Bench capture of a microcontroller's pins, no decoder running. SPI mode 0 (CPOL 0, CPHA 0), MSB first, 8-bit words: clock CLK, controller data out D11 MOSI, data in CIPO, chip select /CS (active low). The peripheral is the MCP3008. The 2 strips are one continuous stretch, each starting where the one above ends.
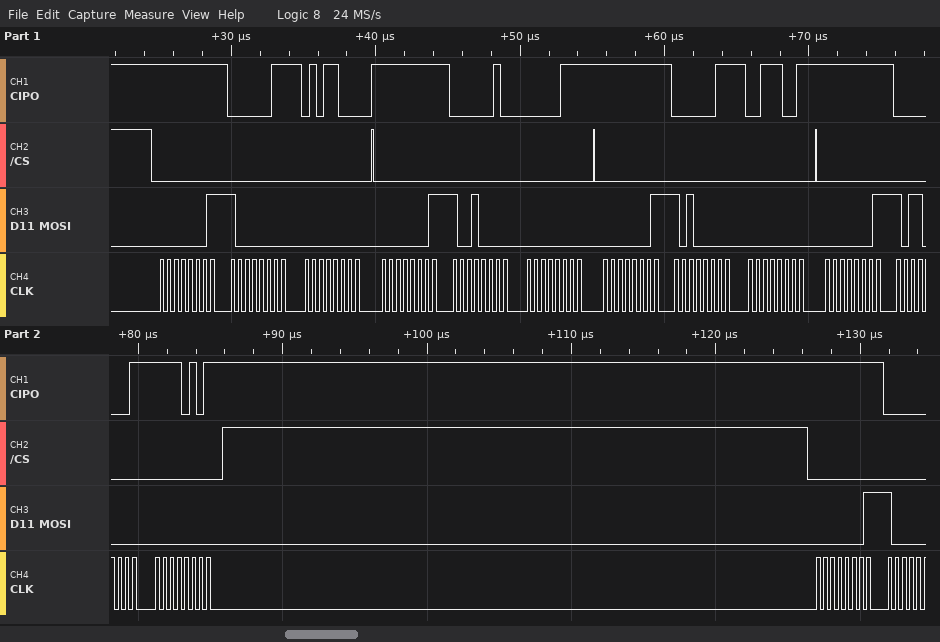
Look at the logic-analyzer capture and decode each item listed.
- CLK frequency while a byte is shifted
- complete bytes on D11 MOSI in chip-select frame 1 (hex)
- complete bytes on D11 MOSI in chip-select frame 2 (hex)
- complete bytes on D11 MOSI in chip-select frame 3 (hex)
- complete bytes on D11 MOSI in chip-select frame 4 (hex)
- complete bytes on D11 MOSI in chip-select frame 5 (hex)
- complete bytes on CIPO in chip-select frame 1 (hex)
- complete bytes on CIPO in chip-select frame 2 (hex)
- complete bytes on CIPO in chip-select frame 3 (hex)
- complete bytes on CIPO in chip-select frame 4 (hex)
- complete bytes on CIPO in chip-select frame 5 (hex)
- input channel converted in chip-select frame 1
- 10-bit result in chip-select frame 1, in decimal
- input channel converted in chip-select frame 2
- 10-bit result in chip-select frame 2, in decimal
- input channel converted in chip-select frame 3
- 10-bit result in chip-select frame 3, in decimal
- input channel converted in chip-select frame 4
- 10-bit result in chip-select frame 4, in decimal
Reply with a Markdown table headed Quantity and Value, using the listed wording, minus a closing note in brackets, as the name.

| Quantity | Value |
|---|---|
| CLK frequency while a byte is shifted | 2 MHz |
| complete bytes on D11 MOSI in chip-select frame 1 | 01 80 00 |
| complete bytes on D11 MOSI in chip-select frame 2 | 01 90 00 |
| complete bytes on D11 MOSI in chip-select frame 3 | 01 A0 00 |
| complete bytes on D11 MOSI in chip-select frame 4 | 01 B0 00 |
| complete bytes on D11 MOSI in chip-select frame 5 | 01 |
| complete bytes on CIPO in chip-select frame 1 | FF 03 58 |
| complete bytes on CIPO in chip-select frame 2 | FF 02 07 |
| complete bytes on CIPO in chip-select frame 3 | FF 03 39 |
| complete bytes on CIPO in chip-select frame 4 | FF 01 F5 |
| complete bytes on CIPO in chip-select frame 5 | FF |
| input channel converted in chip-select frame 1 | 0 |
| 10-bit result in chip-select frame 1, in decimal | 856 |
| input channel converted in chip-select frame 2 | 1 |
| 10-bit result in chip-select frame 2, in decimal | 519 |
| input channel converted in chip-select frame 3 | 2 |
| 10-bit result in chip-select frame 3, in decimal | 825 |
| input channel converted in chip-select frame 4 | 3 |
| 10-bit result in chip-select frame 4, in decimal | 501 |
